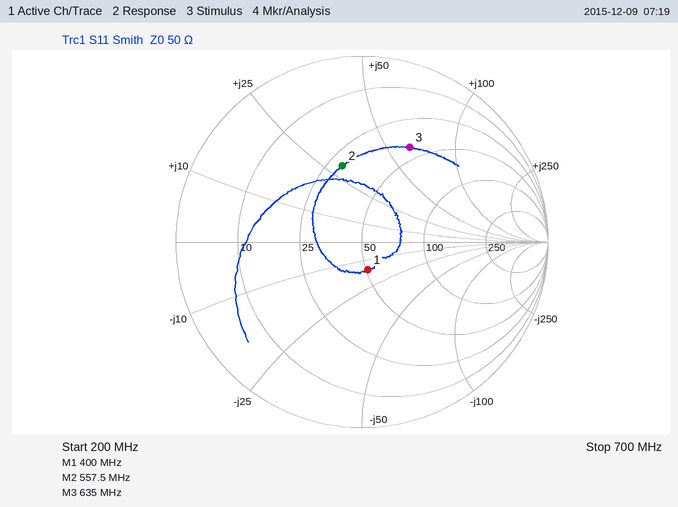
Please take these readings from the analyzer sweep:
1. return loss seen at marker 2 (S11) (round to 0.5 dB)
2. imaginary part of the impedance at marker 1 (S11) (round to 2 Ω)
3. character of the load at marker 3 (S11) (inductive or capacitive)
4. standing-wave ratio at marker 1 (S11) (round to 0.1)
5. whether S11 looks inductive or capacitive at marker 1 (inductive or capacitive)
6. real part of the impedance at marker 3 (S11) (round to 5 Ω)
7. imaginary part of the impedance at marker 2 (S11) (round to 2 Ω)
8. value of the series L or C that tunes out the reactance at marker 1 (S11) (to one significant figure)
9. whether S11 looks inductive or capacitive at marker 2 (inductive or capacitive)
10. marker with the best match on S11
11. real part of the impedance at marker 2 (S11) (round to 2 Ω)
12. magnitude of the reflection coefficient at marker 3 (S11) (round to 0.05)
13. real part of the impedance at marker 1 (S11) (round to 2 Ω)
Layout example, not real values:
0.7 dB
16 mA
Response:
7.5 dB
-16 Ω
inductive
1.4
capacitive
40 Ω
+30 Ω
6 nH
inductive
marker 1
30 Ω
0.55
50 Ω
